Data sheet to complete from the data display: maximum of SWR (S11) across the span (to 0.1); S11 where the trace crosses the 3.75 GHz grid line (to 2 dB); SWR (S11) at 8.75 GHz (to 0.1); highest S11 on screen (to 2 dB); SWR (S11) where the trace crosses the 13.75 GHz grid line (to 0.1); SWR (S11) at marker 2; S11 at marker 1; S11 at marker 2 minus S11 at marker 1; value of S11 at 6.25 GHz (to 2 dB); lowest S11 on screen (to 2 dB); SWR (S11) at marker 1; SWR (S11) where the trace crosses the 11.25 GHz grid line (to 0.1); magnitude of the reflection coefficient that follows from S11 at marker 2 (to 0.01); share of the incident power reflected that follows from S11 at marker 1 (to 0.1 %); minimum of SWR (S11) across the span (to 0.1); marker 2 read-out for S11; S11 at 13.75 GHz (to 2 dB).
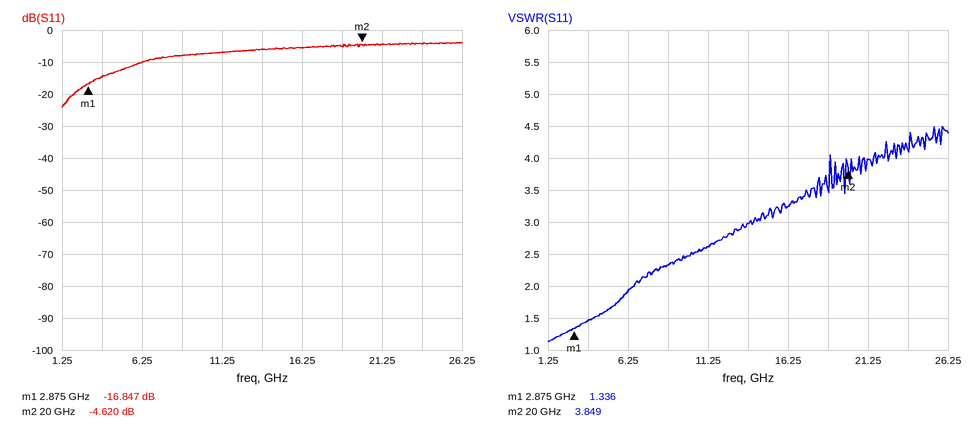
4.5
-14 dB
2.3
-4 dB
3.0
3.849
-16.847 dB
12.227 dB
-10 dB
-24 dB
1.336
2.6
0.59
2.1 %
1.1
-4.620 dB
-6 dB
